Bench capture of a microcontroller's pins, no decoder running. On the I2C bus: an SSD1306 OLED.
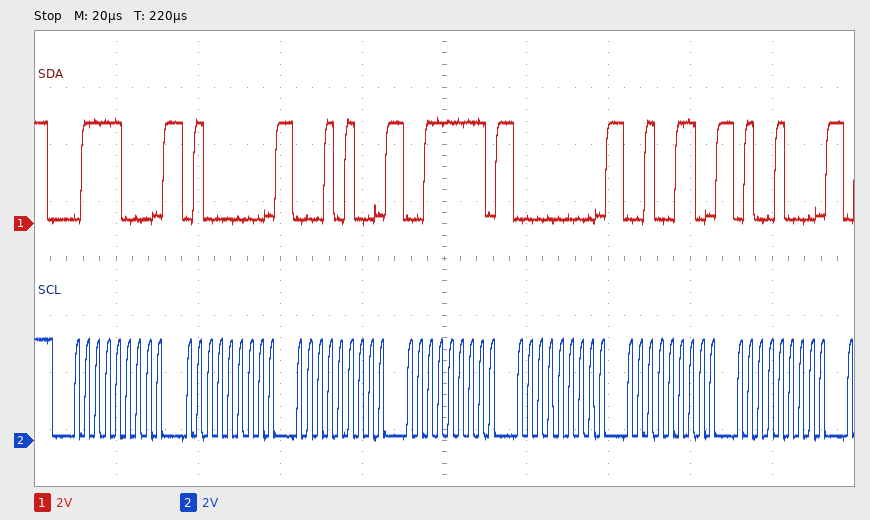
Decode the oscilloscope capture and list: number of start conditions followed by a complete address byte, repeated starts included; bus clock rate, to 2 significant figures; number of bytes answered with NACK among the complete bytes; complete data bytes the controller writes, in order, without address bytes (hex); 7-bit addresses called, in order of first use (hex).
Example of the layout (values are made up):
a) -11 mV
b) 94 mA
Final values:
a) 1
b) 400 kHz
c) 0
d) 40 14 3F 00 26 48
e) 0x3C
